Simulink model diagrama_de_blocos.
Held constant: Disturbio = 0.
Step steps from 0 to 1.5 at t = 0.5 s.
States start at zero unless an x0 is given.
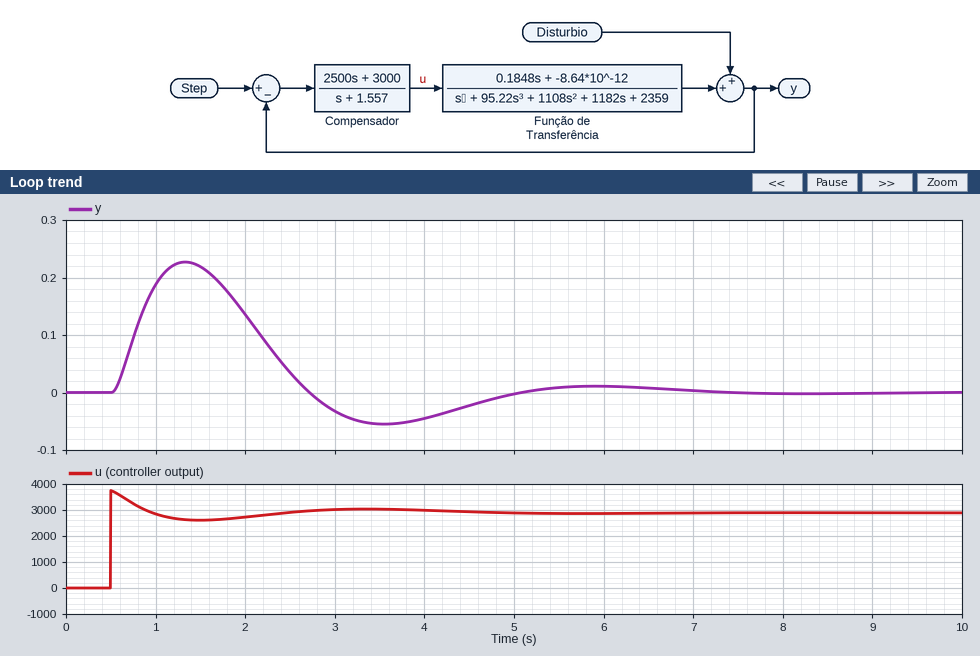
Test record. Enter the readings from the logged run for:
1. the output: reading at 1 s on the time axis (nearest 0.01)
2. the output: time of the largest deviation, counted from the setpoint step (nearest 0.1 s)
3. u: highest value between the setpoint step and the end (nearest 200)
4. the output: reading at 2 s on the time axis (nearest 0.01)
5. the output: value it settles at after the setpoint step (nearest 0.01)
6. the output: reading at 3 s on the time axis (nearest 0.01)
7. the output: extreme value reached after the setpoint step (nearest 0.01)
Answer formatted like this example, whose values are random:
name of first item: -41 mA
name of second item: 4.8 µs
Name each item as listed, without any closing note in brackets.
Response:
the output: reading at 1 s on the time axis: 0.19
the output: time of the largest deviation, counted from the setpoint step: 0.8 s
u: highest value between the setpoint step and the end: 3800
the output: reading at 2 s on the time axis: 0.14
the output: value it settles at after the setpoint step: 0.00
the output: reading at 3 s on the time axis: -0.03
the output: extreme value reached after the setpoint step: 0.23
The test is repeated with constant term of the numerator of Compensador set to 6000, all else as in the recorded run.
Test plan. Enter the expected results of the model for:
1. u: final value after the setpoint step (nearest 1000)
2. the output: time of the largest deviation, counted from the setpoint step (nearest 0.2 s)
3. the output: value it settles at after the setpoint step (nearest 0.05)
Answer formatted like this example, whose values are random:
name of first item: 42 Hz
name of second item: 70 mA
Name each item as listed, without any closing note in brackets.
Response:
u: final value after the setpoint step: 6000
the output: time of the largest deviation, counted from the setpoint step: 1.0 s
the output: value it settles at after the setpoint step: 0.00
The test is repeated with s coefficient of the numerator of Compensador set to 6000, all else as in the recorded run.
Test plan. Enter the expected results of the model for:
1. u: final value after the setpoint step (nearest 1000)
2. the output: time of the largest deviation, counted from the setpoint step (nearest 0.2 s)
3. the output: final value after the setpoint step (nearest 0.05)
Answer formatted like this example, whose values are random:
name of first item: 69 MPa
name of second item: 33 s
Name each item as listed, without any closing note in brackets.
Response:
u: final value after the setpoint step: 3000
the output: time of the largest deviation, counted from the setpoint step: 0.6 s
the output: final value after the setpoint step: 0.00
